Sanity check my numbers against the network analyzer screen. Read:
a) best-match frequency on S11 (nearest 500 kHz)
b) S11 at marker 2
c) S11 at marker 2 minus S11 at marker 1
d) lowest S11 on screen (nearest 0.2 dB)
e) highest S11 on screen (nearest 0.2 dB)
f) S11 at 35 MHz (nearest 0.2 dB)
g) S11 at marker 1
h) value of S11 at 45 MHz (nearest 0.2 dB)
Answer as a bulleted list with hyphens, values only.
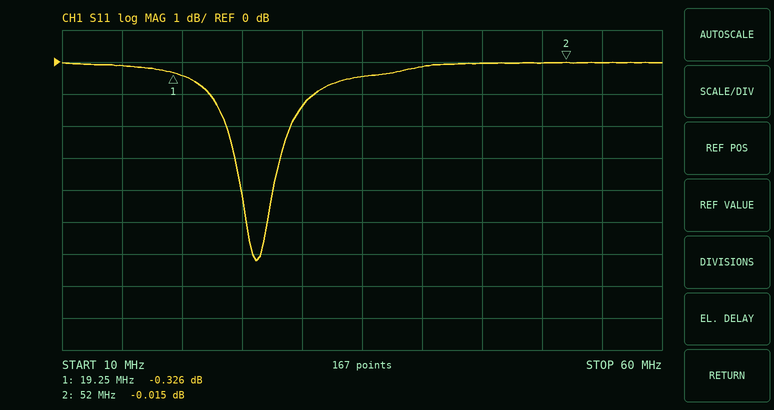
- 26.0 MHz
- -0.015 dB
- 0.311 dB
- -6.2 dB
- 0.0 dB
- -0.4 dB
- -0.326 dB
- 0.0 dB
